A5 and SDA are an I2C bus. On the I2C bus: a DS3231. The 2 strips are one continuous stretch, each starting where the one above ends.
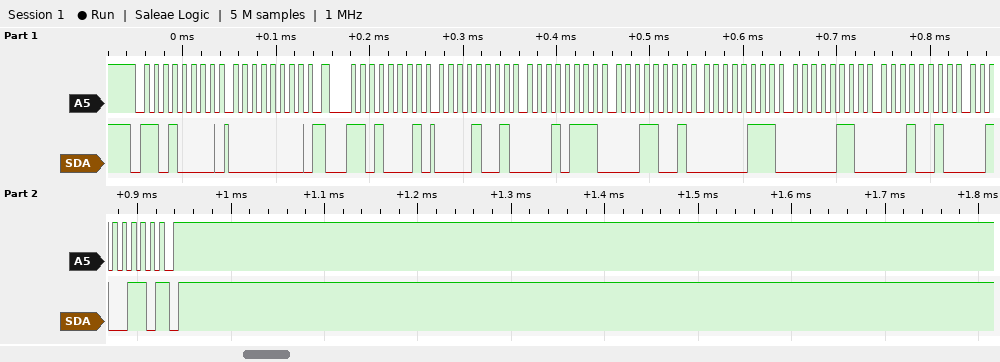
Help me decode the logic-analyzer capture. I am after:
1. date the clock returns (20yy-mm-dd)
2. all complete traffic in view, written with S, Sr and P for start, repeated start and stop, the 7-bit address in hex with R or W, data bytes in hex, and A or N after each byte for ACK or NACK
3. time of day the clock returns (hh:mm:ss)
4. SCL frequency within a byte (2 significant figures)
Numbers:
2026-12-06
S 68W A 00 A Sr 68R A 09 A 17 A 19 A 07 A 06 A 12 A 26 N P
19:17:09
100 kHz
